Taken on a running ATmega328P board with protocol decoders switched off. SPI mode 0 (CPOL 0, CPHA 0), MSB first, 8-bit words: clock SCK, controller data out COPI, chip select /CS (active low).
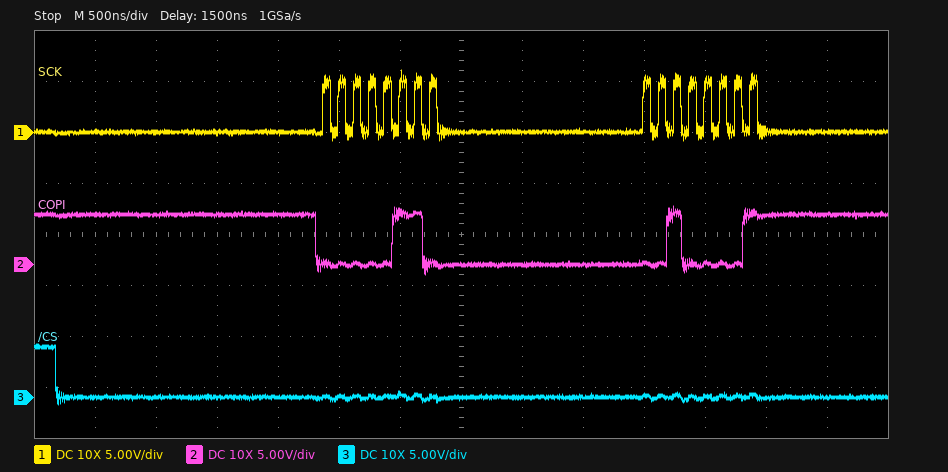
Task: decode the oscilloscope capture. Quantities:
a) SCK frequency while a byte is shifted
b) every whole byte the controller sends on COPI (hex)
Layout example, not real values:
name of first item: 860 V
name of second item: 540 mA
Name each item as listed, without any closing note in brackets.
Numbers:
SCK frequency while a byte is shifted: 8 MHz
every whole byte the controller sends on COPI: 0x06 0x21
